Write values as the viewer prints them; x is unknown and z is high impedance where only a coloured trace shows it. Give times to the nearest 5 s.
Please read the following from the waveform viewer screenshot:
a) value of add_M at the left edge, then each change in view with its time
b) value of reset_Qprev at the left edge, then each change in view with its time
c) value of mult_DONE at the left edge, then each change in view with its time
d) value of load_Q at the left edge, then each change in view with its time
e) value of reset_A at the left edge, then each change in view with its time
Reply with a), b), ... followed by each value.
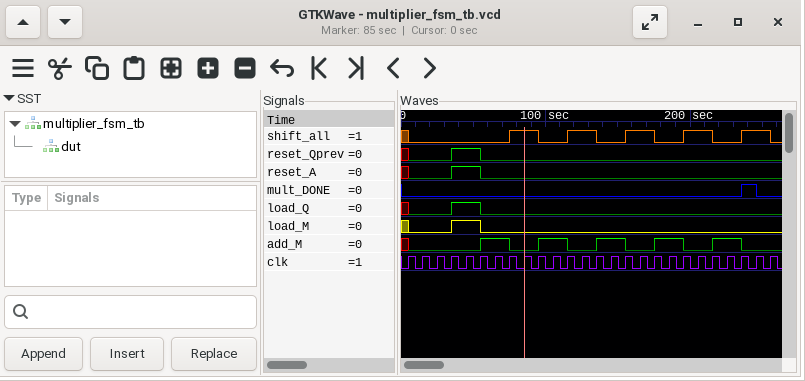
a) x, 0 at 5 s, 1 at 55 s, 0 at 75 s, 1 at 95 s, 0 at 115 s, 1 at 135 s, 0 at 155 s, 1 at 175 s, 0 at 195 s, 1 at 215 s, 0 at 235 s
b) x, 0 at 5 s, 1 at 35 s, 0 at 55 s
c) 0, 1 at 235 s, 0 at 245 s
d) x, 0 at 5 s, 1 at 35 s, 0 at 55 s
e) x, 0 at 5 s, 1 at 35 s, 0 at 55 s
